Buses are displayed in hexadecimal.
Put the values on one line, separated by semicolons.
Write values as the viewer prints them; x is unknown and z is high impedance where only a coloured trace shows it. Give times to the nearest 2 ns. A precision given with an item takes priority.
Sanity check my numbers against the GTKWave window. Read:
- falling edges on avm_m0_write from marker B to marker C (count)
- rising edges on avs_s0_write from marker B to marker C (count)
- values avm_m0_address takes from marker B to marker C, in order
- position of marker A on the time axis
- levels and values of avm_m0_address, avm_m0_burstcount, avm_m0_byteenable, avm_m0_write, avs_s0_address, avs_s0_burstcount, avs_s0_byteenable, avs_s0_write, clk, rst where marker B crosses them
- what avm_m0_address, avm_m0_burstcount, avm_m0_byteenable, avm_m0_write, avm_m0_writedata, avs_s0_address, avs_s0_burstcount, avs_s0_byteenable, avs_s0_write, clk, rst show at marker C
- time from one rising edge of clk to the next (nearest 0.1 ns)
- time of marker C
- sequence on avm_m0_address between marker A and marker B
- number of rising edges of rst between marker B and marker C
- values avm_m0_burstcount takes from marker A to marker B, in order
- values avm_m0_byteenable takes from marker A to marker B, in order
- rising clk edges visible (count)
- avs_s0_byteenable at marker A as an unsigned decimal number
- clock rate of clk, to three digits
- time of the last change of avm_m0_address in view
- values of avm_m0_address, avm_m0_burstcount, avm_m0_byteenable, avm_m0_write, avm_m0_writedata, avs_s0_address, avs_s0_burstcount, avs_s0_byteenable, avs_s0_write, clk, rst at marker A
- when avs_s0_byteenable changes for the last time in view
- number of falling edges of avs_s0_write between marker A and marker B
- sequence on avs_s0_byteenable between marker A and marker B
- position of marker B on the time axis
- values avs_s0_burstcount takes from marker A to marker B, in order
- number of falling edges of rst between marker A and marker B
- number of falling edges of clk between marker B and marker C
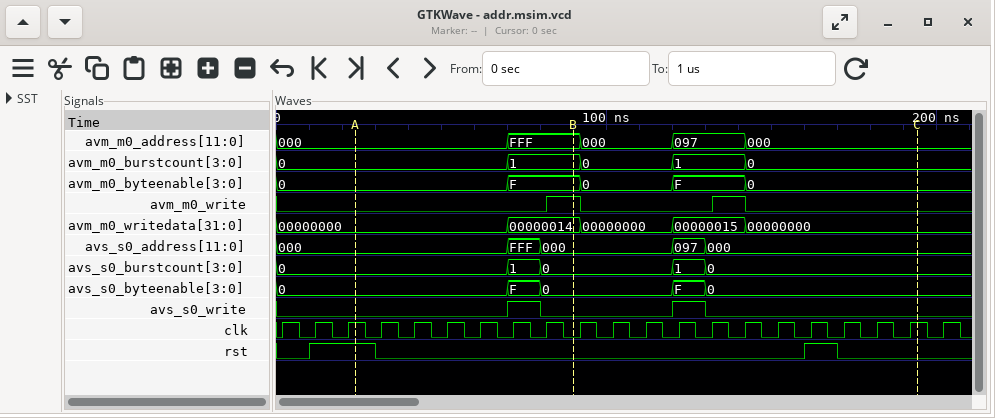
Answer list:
2; 1; FFF, 000, 097, 000; 24 ns; avm_m0_address=FFF, avm_m0_burstcount=1, avm_m0_byteenable=F, avm_m0_write=1, avs_s0_address=000, avs_s0_burstcount=0, avs_s0_byteenable=0, avs_s0_write=0, clk=0, rst=0; avm_m0_address=000, avm_m0_burstcount=0, avm_m0_byteenable=0, avm_m0_write=0, avm_m0_writedata=00000000, avs_s0_address=000, avs_s0_burstcount=0, avs_s0_byteenable=0, avs_s0_write=0, clk=1, rst=0; 10 ns; 194 ns; 000, FFF; 1; 0, 1; 0, F; 21; 0; 100 MHz; 142 ns; avm_m0_address=000, avm_m0_burstcount=0, avm_m0_byteenable=0, avm_m0_write=0, avm_m0_writedata=00000000, avs_s0_address=000, avs_s0_burstcount=0, avs_s0_byteenable=0, avs_s0_write=0, clk=1, rst=1; 130 ns; 1; 0, F, 0; 90 ns; 0, 1, 0; 1; 10
